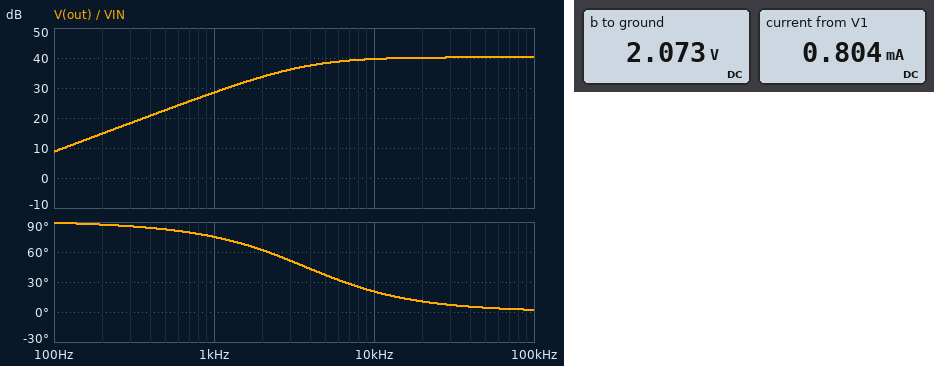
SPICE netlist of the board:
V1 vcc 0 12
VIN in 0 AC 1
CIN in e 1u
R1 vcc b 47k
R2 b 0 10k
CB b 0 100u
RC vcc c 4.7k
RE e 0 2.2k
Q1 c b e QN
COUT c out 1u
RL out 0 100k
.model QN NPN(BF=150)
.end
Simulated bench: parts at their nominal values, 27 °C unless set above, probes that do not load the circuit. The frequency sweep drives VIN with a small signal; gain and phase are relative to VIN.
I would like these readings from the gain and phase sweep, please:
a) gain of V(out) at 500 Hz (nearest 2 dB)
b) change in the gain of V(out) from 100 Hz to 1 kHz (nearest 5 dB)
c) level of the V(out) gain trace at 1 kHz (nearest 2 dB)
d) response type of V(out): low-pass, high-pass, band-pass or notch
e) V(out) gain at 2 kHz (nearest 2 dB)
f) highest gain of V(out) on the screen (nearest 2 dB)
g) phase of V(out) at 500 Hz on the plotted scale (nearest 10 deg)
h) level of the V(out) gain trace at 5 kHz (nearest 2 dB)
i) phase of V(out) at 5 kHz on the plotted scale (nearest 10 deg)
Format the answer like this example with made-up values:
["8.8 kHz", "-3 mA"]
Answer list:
["22 dB", "20 dB", "28 dB", "high-pass", "34 dB", "40 dB", "80 deg", "38 dB", "40 deg"]
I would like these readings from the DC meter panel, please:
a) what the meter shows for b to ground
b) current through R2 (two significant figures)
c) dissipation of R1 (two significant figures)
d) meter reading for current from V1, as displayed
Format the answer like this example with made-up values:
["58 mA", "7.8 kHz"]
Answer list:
["2.073 V", "210 µA", "2.1 mW", "0.804 mA"]
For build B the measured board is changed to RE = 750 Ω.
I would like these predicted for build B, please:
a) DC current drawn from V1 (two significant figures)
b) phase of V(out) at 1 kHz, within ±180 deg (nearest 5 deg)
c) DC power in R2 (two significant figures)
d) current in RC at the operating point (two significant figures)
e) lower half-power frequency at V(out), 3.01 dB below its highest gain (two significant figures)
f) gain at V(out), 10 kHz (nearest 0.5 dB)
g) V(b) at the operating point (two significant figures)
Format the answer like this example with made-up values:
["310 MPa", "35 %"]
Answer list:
["1.8 mA", "85 deg", "410 µW", "1.6 mA", "10 kHz", "46.0 dB", "2.0 V"]
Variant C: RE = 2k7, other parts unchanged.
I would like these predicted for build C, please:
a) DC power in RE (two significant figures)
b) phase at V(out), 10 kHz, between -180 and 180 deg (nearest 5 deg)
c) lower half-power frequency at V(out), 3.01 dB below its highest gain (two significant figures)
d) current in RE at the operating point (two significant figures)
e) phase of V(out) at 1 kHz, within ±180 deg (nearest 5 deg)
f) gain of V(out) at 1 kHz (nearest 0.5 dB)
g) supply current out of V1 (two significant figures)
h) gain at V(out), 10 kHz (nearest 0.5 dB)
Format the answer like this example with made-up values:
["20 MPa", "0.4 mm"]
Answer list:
["650 µW", "15 deg", "3.1 kHz", "490 µA", "70 deg", "28.5 dB", "700 µA", "38.0 dB"]
